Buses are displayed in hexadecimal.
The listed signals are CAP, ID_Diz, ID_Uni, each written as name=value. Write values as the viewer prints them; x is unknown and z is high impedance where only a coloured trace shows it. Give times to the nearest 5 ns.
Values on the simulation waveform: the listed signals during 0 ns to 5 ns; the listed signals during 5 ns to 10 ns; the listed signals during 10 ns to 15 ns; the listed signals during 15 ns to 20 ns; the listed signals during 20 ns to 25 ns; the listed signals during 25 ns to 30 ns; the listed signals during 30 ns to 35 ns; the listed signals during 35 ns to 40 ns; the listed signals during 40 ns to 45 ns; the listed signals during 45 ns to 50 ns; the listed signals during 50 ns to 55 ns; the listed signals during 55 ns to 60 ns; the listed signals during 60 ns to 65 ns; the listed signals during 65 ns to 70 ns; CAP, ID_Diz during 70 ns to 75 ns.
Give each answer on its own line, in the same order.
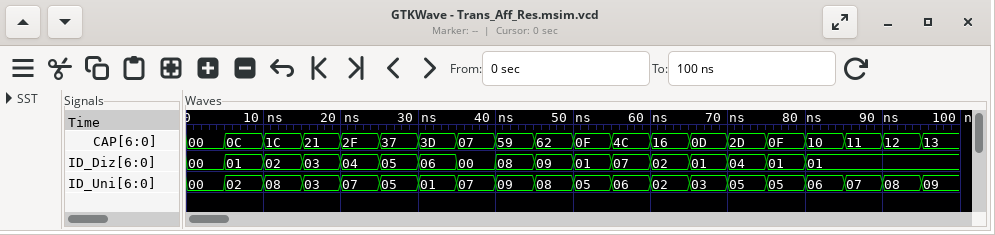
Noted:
CAP=00, ID_Diz=00, ID_Uni=00
CAP=0C, ID_Diz=01, ID_Uni=02
CAP=1C, ID_Diz=02, ID_Uni=08
CAP=21, ID_Diz=03, ID_Uni=03
CAP=2F, ID_Diz=04, ID_Uni=07
CAP=37, ID_Diz=05, ID_Uni=05
CAP=3D, ID_Diz=06, ID_Uni=01
CAP=07, ID_Diz=00, ID_Uni=07
CAP=59, ID_Diz=08, ID_Uni=09
CAP=62, ID_Diz=09, ID_Uni=08
CAP=0F, ID_Diz=01, ID_Uni=05
CAP=4C, ID_Diz=07, ID_Uni=06
CAP=16, ID_Diz=02, ID_Uni=02
CAP=0D, ID_Diz=01, ID_Uni=03
CAP=2D, ID_Diz=04
